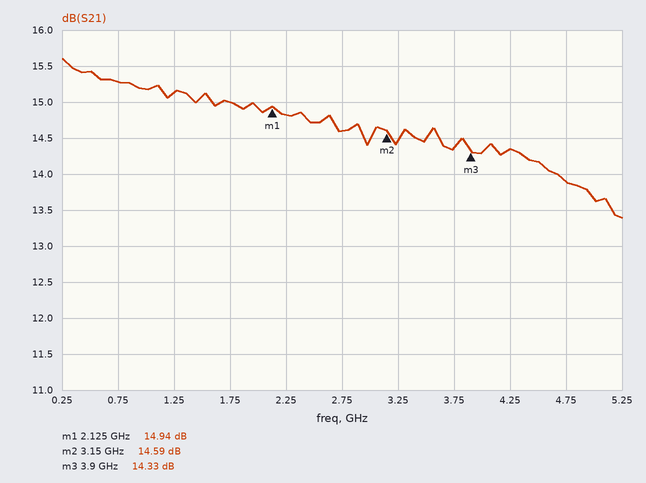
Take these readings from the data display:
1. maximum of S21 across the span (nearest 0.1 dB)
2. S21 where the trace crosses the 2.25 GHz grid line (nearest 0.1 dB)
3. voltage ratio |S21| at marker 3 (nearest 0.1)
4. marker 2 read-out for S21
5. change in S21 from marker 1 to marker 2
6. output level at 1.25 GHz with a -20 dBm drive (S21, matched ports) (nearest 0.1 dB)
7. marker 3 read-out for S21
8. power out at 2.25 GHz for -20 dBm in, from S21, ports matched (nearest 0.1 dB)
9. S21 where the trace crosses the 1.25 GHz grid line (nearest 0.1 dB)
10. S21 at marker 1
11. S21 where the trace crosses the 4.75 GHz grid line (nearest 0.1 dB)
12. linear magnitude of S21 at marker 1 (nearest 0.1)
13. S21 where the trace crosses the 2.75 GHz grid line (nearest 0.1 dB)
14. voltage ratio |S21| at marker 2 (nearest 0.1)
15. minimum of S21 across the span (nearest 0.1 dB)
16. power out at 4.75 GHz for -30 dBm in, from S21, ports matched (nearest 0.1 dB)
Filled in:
15.6 dB
14.8 dB
5.2
14.59 dB
-0.35 dB
-4.9 dBm
14.33 dB
-5.2 dBm
15.1 dB
14.94 dB
13.9 dB
5.6
14.6 dB
5.4
13.4 dB
-16.1 dBm
